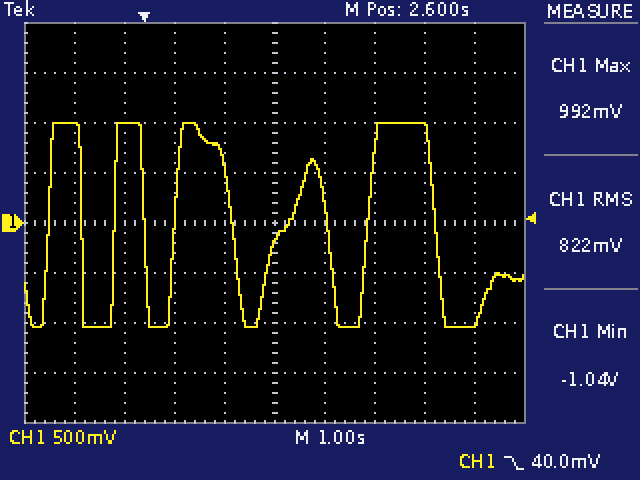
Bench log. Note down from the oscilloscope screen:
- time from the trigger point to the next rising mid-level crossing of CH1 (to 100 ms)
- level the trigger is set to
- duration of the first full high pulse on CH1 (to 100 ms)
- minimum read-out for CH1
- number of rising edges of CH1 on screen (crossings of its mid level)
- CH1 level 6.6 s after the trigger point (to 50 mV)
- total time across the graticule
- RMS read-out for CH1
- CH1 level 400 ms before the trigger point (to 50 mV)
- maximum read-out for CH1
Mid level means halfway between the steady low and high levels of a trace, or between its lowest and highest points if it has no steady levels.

600 ms
40.0 mV
700 ms
-1.04 V
5
-1.00 V
10 s
822 mV
1.00 V
992 mV
